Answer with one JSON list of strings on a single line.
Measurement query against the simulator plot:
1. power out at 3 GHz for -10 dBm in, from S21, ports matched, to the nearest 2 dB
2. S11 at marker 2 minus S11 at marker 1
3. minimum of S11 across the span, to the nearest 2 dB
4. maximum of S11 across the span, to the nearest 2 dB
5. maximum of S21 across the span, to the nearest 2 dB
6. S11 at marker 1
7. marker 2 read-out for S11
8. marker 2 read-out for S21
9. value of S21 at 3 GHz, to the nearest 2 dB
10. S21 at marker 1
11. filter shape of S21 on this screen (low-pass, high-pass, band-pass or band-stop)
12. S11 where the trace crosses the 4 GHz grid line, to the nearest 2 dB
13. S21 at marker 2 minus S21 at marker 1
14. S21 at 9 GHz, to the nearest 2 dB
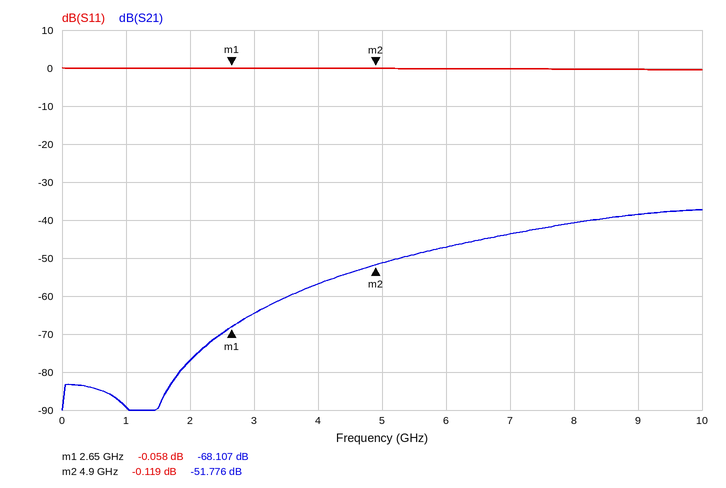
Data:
["-74 dBm", "-0.061 dB", "0 dB", "0 dB", "-38 dB", "-0.058 dB", "-0.119 dB", "-51.776 dB", "-64 dB", "-68.107 dB", "high-pass", "0 dB", "16.331 dB", "-38 dB"]
